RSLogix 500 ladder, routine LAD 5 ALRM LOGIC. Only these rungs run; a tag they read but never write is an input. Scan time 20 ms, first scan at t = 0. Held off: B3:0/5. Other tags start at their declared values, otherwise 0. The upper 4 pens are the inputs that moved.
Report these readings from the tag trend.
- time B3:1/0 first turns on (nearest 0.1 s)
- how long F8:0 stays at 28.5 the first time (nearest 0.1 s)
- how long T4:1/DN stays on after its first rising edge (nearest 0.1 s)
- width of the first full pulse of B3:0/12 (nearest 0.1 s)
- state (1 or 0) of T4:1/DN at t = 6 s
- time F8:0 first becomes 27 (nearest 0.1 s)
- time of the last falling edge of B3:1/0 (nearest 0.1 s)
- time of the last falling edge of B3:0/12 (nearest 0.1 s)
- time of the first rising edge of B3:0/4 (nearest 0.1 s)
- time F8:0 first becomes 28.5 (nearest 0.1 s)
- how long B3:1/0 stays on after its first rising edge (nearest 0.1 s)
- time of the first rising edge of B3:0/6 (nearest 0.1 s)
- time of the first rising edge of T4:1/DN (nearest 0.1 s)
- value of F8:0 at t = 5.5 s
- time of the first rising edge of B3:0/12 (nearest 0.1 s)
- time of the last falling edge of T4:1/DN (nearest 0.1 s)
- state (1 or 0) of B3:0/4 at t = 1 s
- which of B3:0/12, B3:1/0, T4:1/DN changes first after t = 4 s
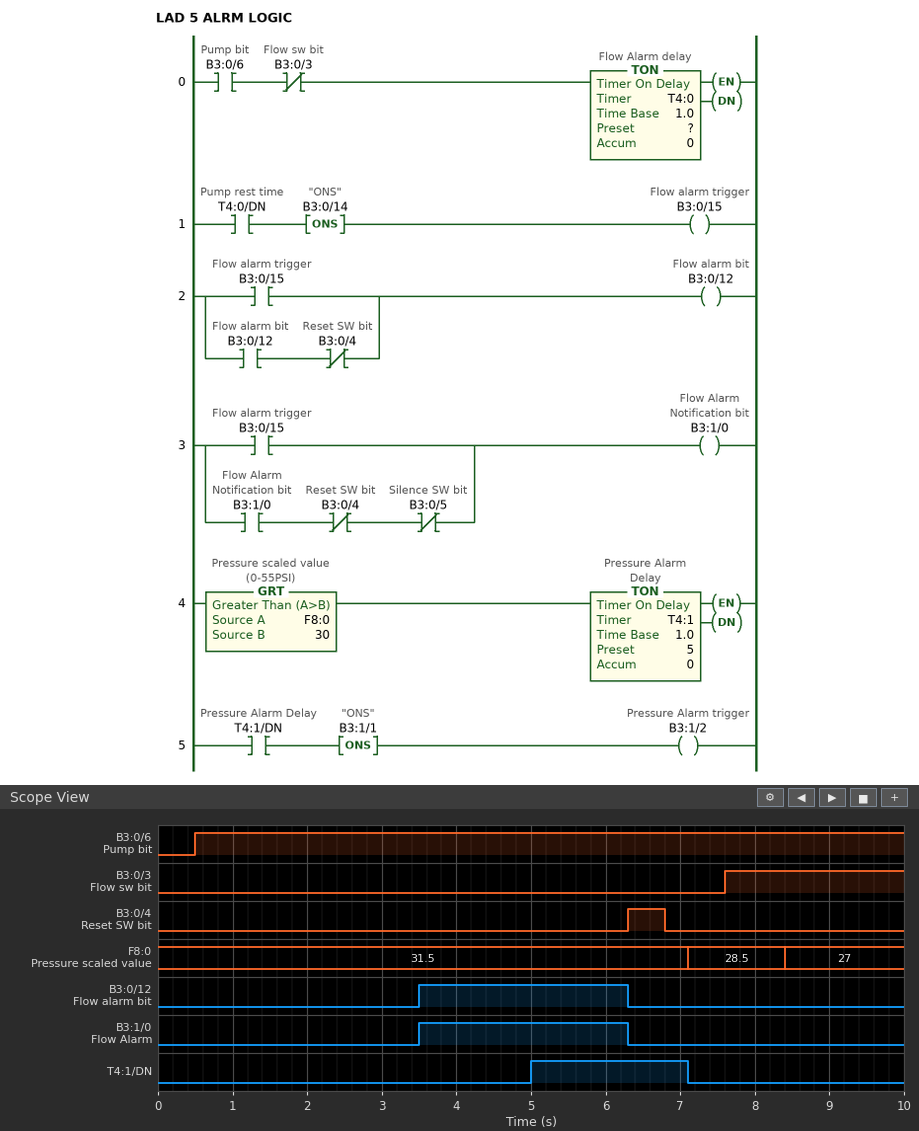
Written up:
3.5 s
1.3 s
2.1 s
2.8 s
1
8.4 s
6.3 s
6.3 s
6.3 s
7.1 s
2.8 s
0.5 s
5.0 s
31.5
3.5 s
7.1 s
0
T4:1/DN
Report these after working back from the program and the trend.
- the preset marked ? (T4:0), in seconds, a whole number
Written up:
3 s
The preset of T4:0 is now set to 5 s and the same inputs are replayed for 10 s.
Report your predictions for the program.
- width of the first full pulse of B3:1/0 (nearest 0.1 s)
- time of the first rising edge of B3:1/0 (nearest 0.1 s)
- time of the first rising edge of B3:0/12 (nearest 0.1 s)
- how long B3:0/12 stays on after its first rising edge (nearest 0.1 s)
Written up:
0.8 s
5.5 s
5.5 s
0.8 s
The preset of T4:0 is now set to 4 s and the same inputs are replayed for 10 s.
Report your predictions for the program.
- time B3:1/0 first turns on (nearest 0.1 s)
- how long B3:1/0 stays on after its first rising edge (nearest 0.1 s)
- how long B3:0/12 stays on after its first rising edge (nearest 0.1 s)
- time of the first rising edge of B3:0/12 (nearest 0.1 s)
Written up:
4.5 s
1.8 s
1.8 s
4.5 s
